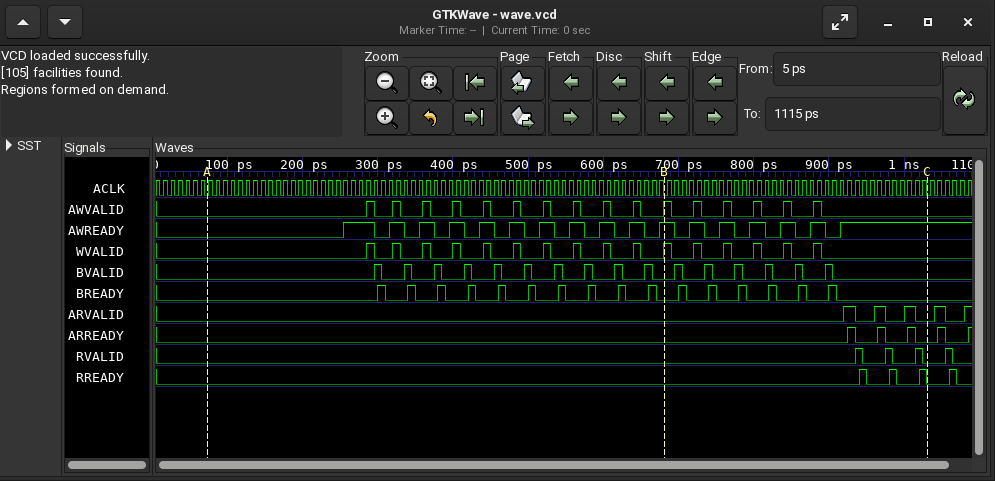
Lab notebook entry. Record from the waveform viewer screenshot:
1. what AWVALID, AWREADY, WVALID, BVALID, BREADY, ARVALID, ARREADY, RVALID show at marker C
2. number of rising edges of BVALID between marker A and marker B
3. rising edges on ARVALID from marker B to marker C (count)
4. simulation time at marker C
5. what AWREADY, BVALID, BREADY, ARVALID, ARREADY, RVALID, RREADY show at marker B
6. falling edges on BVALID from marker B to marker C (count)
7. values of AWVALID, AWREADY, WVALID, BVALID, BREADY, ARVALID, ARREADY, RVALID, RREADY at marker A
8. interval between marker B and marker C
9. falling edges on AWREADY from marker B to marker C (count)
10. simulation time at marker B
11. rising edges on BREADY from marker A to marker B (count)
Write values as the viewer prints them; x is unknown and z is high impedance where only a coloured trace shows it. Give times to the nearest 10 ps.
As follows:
AWVALID=0, AWREADY=1, WVALID=0, BVALID=0, BREADY=0, ARVALID=0, ARREADY=0, RVALID=0
10
3
1030 ps
AWREADY=1, BVALID=0, BREADY=0, ARVALID=0, ARREADY=0, RVALID=0, RREADY=0
6
AWVALID=0, AWREADY=0, WVALID=0, BVALID=0, BREADY=0, ARVALID=0, ARREADY=0, RVALID=0, RREADY=0
350 ps
6
680 ps
10
